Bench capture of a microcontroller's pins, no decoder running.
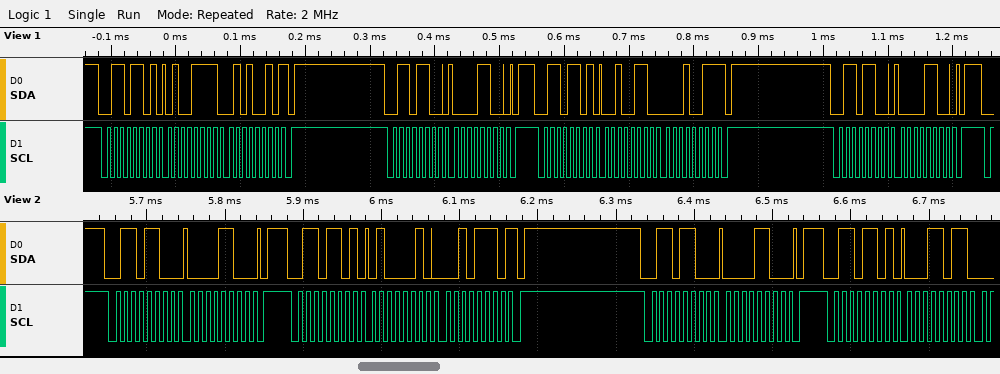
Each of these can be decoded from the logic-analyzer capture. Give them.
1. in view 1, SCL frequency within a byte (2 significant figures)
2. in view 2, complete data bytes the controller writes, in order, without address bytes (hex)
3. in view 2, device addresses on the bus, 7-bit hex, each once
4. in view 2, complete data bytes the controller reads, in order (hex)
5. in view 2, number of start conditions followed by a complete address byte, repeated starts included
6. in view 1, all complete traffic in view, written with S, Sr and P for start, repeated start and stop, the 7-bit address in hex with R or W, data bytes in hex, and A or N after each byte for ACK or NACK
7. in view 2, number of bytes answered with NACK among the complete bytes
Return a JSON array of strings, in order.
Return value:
["100 kHz", "0C 0C", "0x36", "42 2E 1B", "4", "S 36R A 4F A 52 N P S 36W A 0C A P S 36R A 26 A 13 N P S 36W A 0C A P", "1"]
